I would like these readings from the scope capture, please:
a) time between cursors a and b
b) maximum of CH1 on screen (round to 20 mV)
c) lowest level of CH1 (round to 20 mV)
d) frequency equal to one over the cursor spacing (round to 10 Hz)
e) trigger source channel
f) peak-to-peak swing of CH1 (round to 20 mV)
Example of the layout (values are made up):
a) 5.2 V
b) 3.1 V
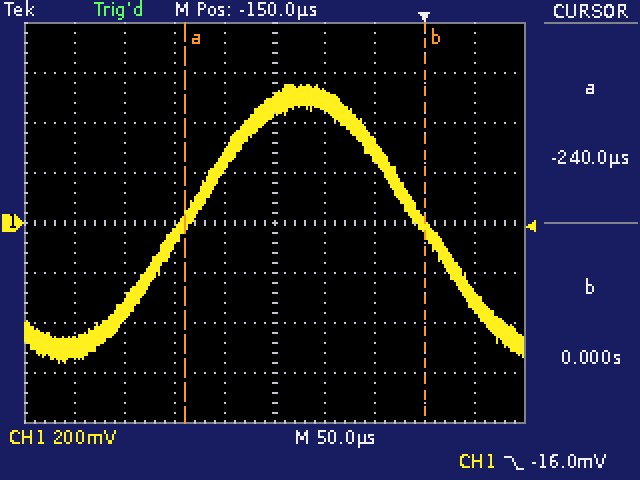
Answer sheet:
a) 240 µs
b) 560 mV
c) -560 mV
d) 4.17 kHz
e) CH1
f) 1.12 V
